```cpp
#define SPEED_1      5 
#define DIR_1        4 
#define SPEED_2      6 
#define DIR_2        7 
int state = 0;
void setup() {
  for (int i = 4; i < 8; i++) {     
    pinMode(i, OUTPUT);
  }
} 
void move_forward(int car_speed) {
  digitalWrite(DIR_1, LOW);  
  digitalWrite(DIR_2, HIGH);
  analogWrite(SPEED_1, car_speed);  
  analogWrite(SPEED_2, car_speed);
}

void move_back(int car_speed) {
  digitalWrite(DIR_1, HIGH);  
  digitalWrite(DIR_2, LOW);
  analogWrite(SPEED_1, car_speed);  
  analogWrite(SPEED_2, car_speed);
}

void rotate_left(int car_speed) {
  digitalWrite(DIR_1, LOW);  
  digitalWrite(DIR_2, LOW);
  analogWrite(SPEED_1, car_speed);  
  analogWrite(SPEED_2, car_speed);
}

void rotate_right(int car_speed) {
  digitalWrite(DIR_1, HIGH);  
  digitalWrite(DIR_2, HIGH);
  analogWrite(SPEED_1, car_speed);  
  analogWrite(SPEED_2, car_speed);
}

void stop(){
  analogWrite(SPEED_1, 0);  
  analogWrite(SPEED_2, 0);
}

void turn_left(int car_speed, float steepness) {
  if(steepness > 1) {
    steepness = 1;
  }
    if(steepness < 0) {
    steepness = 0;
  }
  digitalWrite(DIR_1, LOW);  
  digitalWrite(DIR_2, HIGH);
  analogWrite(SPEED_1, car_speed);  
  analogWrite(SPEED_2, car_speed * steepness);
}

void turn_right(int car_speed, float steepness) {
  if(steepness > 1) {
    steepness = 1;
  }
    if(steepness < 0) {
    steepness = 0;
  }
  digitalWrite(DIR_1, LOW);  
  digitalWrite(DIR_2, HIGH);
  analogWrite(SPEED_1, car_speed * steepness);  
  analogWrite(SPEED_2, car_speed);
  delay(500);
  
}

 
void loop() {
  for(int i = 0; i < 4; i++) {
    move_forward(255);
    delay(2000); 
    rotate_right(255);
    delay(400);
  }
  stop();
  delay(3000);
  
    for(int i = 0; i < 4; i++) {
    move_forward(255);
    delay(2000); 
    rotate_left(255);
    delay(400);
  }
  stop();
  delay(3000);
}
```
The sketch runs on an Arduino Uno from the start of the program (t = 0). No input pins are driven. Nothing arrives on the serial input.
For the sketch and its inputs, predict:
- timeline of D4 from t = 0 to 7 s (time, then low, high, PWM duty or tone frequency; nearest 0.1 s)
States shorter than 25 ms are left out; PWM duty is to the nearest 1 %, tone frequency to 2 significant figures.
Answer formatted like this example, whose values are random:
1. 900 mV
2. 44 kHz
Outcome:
1. 0 s low; 2 s high; 2.4 s low; 4.4 s high; 4.8 s low; 6.8 s high
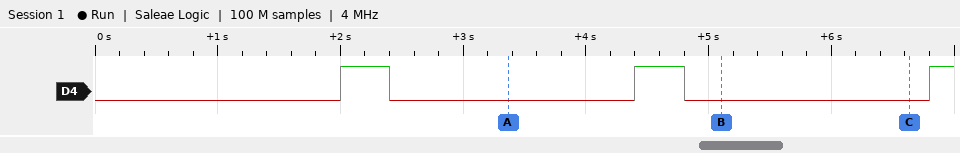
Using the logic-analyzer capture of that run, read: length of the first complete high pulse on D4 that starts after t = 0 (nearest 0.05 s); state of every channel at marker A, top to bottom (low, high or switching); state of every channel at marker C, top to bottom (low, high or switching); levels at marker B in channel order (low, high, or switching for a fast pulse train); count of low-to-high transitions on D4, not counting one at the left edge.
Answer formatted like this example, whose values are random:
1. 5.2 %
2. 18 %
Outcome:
1. 0.40 s
2. D4 low
3. D4 low
4. D4 low
5. 3
